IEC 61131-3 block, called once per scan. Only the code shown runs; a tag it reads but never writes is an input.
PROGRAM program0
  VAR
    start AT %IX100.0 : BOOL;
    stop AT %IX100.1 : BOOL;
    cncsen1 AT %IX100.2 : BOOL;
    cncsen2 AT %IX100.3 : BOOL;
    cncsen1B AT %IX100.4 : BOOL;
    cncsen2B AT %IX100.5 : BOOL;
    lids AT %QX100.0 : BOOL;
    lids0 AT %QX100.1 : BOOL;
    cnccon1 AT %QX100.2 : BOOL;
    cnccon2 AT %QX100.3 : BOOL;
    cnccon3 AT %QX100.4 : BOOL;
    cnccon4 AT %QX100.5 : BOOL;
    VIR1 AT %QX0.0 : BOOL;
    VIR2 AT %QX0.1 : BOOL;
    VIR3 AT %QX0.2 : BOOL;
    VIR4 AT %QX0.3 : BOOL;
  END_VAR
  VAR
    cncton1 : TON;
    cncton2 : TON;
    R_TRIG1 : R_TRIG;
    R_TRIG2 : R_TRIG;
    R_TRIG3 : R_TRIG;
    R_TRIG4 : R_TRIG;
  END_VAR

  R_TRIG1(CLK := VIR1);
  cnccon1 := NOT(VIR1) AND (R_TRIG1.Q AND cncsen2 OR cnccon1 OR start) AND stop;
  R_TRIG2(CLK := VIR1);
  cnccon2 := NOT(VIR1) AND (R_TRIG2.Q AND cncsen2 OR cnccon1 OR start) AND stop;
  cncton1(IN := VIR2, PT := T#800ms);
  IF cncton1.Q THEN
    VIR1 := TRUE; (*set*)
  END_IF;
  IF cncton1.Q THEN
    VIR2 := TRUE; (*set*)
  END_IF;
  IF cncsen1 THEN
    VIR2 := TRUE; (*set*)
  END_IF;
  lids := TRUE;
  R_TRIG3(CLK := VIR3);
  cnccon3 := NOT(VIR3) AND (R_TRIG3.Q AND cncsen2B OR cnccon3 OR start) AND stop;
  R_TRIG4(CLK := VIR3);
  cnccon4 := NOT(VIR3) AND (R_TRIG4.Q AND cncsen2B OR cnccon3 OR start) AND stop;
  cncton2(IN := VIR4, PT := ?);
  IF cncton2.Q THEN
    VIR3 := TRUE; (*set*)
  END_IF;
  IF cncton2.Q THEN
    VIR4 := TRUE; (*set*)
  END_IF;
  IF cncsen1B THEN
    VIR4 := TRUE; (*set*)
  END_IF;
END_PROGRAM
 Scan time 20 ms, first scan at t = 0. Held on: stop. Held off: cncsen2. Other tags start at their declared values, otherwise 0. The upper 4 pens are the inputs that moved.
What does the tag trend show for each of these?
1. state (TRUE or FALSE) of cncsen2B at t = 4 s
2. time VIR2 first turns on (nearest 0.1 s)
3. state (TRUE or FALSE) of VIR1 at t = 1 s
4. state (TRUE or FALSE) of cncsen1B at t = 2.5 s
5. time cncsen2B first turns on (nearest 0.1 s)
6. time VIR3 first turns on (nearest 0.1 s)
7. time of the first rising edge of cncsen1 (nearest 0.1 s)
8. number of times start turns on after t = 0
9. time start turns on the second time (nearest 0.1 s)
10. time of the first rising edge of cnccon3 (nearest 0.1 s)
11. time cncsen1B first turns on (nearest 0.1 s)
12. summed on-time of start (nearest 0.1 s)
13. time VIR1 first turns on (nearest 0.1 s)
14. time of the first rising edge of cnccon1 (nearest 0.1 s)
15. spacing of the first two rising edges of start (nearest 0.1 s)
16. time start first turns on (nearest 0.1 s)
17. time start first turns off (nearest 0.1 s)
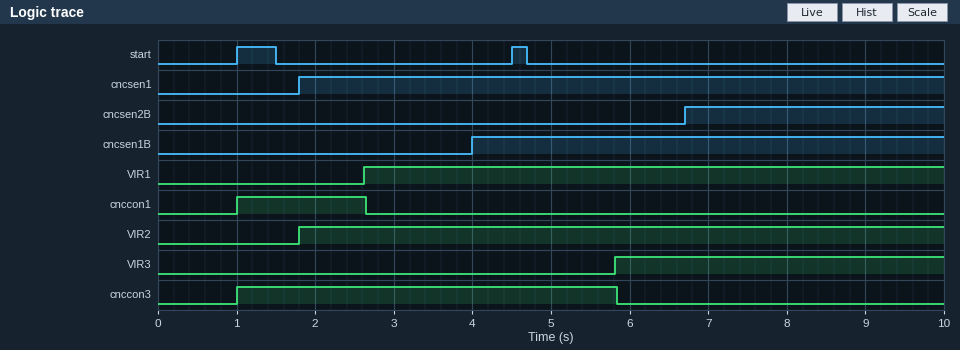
FALSE
1.8 s
FALSE
FALSE
6.7 s
5.8 s
1.8 s
2
4.5 s
1.0 s
4.0 s
0.7 s
2.6 s
1.0 s
3.5 s
1.0 s
1.5 s
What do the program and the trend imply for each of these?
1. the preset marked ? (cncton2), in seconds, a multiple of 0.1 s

1.8 s
